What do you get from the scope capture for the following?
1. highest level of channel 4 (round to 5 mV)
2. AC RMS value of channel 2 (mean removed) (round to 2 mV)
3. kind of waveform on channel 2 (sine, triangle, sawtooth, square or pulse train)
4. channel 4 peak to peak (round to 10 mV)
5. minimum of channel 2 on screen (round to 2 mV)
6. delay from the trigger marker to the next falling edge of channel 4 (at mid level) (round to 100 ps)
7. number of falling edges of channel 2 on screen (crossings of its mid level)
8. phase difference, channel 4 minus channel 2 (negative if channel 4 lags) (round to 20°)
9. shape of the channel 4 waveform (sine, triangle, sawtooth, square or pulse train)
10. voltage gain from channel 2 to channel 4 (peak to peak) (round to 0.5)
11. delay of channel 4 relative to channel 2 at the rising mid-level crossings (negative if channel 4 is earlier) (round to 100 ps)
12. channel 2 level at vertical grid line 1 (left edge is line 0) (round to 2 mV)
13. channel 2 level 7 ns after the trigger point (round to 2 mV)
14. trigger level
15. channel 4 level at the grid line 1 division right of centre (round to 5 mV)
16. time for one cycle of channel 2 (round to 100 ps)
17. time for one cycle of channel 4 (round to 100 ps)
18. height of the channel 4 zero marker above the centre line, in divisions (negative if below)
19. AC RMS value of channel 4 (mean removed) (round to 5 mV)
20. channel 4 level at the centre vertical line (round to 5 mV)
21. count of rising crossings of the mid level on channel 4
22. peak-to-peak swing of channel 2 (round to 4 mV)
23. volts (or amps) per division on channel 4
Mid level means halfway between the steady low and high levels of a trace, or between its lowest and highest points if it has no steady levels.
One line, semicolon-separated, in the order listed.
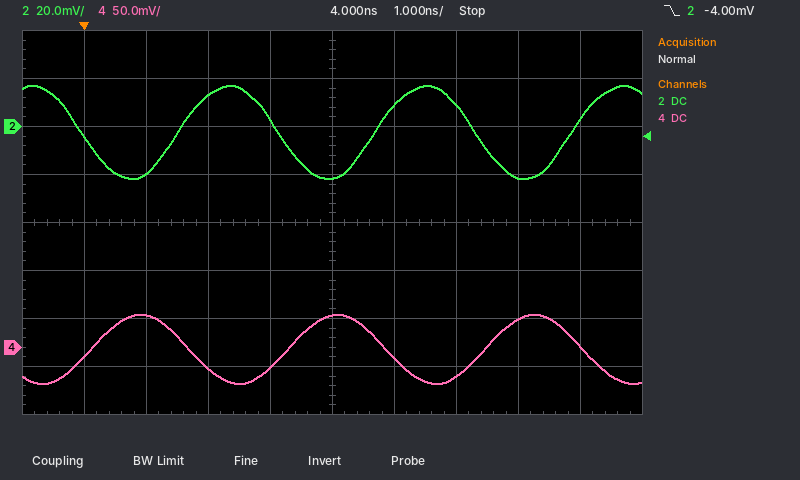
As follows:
35 mV; 14 mV; sine; 70 mV; -22 mV; 1.7 ns; 3; +160°; sine; 2.0; -1.4 ns; -4 mV; -22 mV; -4.00 mV; -10 mV; 3.2 ns; 3.2 ns; -2.6 div; 25 mV; 35 mV; 3; 40 mV; 50 mV
